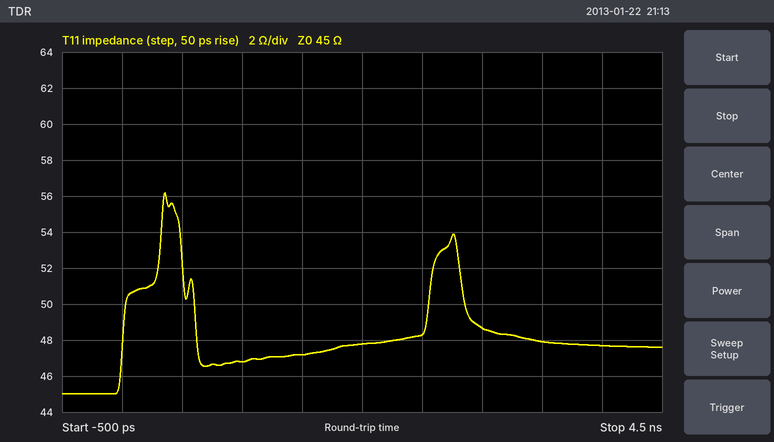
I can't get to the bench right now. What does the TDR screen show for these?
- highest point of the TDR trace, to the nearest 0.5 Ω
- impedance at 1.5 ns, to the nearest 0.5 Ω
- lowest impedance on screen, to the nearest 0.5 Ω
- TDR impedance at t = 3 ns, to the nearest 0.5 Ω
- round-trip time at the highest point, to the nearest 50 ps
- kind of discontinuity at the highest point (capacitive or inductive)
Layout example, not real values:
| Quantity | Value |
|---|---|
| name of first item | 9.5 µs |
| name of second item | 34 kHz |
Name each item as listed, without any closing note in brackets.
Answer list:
| Quantity | Value |
|---|---|
| highest point of the TDR trace, to the nearest 0.5 Ω | 56.0 Ω |
| impedance at 1.5 ns, to the nearest 0.5 Ω | 47.0 Ω |
| lowest impedance on screen, to the nearest 0.5 Ω | 45.0 Ω |
| TDR impedance at t = 3 ns, to the nearest 0.5 Ω | 48.5 Ω |
| round-trip time at the highest point, to the nearest 50 ps | 350 ps |
| kind of discontinuity at the highest point | inductive |
